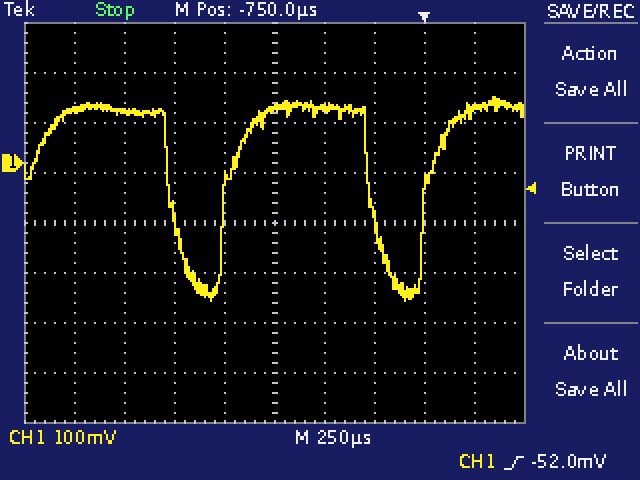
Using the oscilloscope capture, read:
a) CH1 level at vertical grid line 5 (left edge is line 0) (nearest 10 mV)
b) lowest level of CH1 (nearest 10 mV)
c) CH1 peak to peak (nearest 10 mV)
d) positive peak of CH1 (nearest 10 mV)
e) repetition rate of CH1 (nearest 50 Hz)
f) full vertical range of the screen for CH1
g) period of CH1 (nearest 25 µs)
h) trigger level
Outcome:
110 mV
-280 mV
410 mV
130 mV
1.00 kHz
800 mV
1.000 ms
-52.0 mV
